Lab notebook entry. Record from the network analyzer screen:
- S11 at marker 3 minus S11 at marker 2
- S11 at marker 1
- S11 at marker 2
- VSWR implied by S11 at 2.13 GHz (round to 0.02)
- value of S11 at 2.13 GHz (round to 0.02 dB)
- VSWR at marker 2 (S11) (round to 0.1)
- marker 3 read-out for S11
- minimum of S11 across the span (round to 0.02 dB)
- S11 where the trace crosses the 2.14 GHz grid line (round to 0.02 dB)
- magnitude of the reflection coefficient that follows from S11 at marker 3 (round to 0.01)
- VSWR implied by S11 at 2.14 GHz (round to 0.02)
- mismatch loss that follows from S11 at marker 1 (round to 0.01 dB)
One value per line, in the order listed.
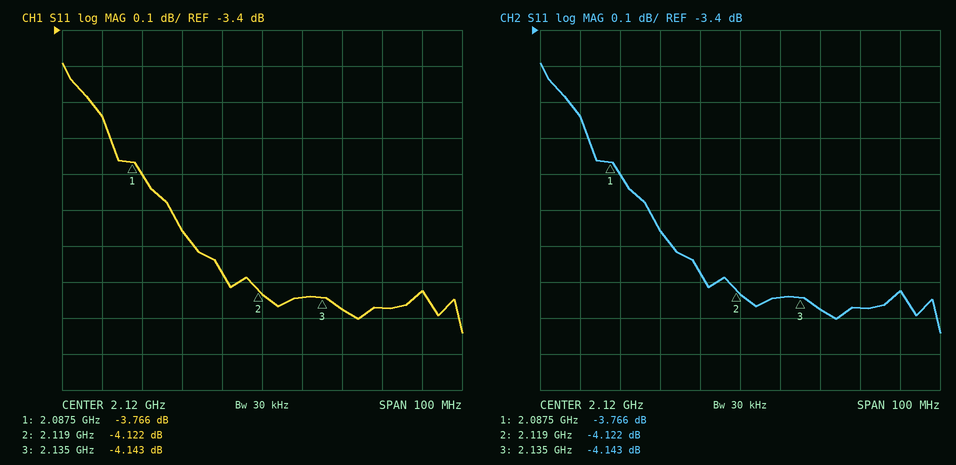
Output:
-0.021 dB
-3.766 dB
-4.122 dB
4.28
-4.14 dB
4.3
-4.143 dB
-4.24 dB
-4.18 dB
0.62
4.24
2.37 dB
